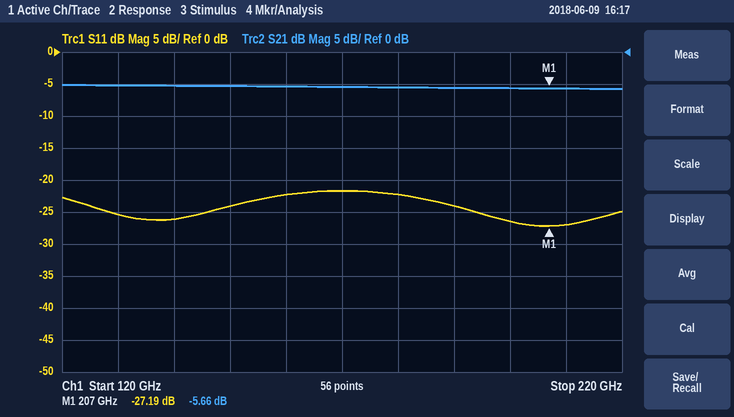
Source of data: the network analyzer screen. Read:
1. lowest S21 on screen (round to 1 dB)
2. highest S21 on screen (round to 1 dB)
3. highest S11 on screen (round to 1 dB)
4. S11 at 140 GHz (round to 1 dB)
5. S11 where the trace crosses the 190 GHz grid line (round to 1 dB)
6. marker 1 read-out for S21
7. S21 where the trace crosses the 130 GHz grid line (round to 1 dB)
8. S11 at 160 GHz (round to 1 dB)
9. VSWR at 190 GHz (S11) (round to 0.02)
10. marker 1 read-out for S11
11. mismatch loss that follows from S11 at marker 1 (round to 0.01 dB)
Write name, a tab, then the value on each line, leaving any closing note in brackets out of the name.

lowest S21 on screen	-6 dB
highest S21 on screen	-5 dB
highest S11 on screen	-22 dB
S11 at 140 GHz	-26 dB
S11 where the trace crosses the 190 GHz grid line	-24 dB
marker 1 read-out for S21	-5.66 dB
S21 where the trace crosses the 130 GHz grid line	-5 dB
S11 at 160 GHz	-22 dB
VSWR at 190 GHz (S11)	1.14
marker 1 read-out for S11	-27.19 dB
mismatch loss that follows from S11 at marker 1	0.01 dB
